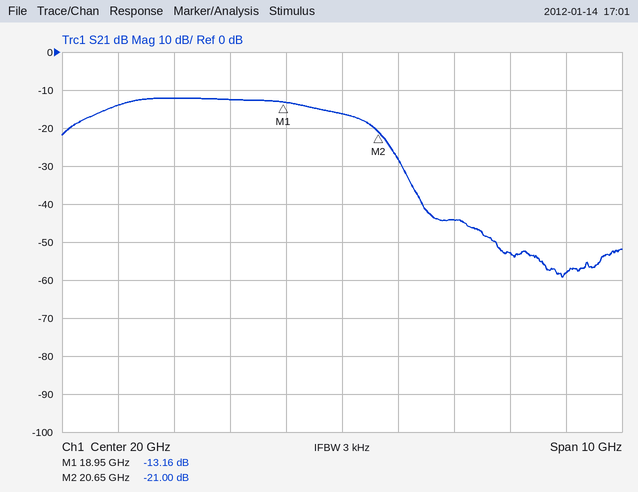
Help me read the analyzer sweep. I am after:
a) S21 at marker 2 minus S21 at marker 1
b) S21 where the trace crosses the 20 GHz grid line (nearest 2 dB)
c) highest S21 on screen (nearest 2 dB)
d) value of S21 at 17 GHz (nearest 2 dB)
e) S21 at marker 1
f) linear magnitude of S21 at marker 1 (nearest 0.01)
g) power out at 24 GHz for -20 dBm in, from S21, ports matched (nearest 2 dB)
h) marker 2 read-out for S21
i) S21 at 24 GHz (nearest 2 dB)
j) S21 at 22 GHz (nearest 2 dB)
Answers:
-7.84 dB
-16 dB
-12 dB
-12 dB
-13.16 dB
0.22
-78 dBm
-21.00 dB
-58 dB
-44 dB
